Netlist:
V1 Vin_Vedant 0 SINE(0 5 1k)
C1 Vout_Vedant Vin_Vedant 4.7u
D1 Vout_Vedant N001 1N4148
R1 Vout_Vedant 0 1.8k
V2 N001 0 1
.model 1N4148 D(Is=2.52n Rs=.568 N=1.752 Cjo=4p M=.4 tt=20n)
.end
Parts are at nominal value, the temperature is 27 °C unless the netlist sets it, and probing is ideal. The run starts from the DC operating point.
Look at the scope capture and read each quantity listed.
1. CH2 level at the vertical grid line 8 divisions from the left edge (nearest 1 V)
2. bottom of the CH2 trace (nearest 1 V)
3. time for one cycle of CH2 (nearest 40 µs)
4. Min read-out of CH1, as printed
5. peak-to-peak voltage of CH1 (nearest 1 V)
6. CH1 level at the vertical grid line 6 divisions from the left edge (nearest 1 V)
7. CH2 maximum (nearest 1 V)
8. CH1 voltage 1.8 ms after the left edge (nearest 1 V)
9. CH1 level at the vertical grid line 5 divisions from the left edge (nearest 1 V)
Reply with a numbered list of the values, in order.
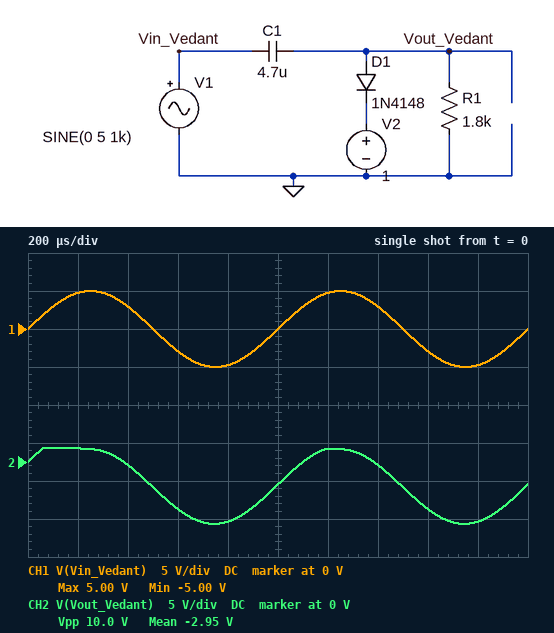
1. -6 V
2. -8 V
3. 1.00 ms
4. -5.00 V
5. 10 V
6. 5 V
7. 2 V
8. -5 V
9. 0 V
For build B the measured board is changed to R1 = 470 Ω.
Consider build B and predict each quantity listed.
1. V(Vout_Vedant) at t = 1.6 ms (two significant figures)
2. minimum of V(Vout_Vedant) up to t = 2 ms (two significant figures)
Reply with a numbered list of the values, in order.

1. -6.0 V
2. -7.6 V
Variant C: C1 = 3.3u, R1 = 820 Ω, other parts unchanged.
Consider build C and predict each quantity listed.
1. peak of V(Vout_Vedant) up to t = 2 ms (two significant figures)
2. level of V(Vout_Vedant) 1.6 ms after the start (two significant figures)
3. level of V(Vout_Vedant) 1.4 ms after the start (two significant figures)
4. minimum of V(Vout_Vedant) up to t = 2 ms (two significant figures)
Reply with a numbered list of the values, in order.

1. 1.8 V
2. -6.1 V
3. -460 mV
4. -7.8 V
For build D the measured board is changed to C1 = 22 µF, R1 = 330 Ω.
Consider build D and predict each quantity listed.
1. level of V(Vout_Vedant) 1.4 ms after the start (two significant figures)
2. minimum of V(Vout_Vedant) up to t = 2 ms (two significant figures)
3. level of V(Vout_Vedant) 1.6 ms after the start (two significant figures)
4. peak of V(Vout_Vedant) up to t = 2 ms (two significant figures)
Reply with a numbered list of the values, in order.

1. -310 mV
2. -8.0 V
3. -6.1 V
4. 2.2 V
